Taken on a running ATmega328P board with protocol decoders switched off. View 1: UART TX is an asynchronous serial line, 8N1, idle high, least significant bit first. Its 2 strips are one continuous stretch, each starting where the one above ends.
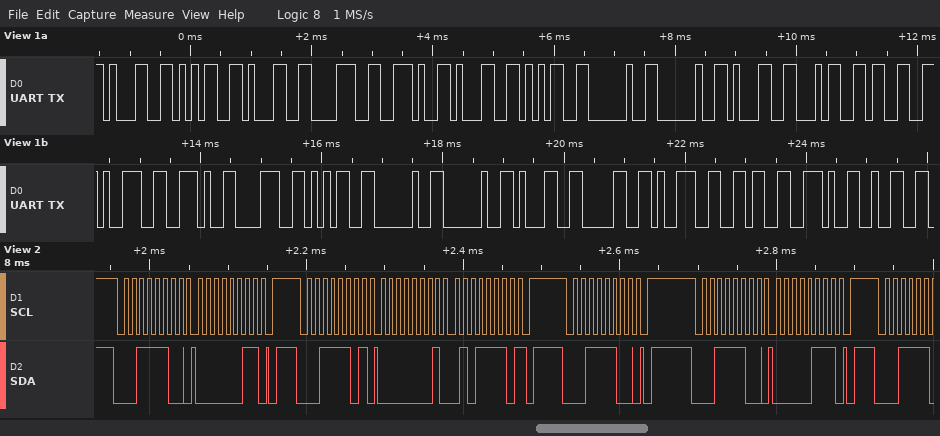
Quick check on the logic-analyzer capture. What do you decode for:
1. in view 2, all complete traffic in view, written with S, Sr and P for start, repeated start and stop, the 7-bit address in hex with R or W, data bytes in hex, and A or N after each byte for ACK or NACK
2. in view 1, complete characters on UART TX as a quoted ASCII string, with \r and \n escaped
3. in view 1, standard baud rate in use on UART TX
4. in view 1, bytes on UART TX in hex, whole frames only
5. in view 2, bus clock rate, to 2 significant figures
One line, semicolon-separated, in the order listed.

S 1EW A 03 A P S 1ER A 01 A 5E N P S 1EW A P S 1EW A 07 A P; "1518.15  1439.85  1096.2"; 9600 baud; 31 35 31 38 2E 31 35 20 20 31 34 33 39 2E 38 35 20 20 31 30 39 36 2E 32; 100 kHz
